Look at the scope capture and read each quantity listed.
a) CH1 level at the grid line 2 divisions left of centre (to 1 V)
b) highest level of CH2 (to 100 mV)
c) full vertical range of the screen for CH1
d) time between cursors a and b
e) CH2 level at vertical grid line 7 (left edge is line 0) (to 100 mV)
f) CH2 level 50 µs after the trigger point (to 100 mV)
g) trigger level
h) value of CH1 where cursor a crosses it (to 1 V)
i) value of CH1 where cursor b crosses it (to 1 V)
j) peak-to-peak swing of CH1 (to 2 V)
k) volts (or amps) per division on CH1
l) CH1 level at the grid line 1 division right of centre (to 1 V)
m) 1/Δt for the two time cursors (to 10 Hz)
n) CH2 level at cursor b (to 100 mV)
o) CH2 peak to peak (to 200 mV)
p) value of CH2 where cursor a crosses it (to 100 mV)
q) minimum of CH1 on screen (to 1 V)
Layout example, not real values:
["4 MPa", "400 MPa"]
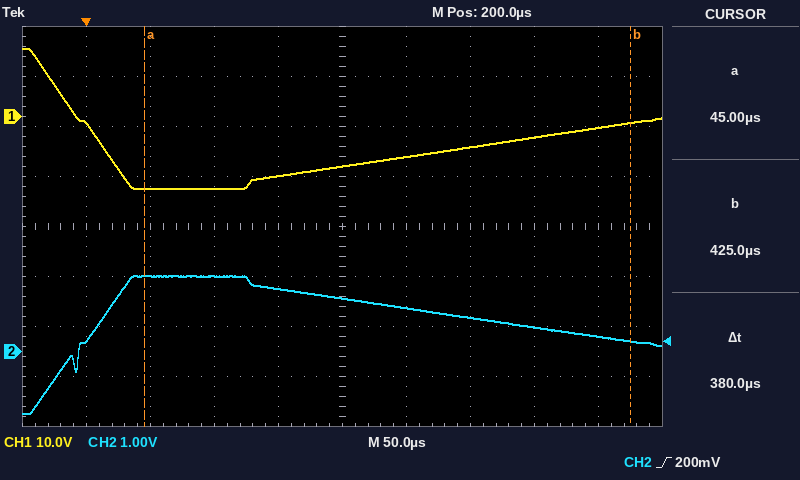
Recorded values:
["-14 V", "1.5 V", "80 V", "380 µs", "700 mV", "1.5 V", "200 mV", "-14 V", "-1 V", "28 V", "10 V", "-8 V", "2.63 kHz", "200 mV", "2.8 V", "1.5 V", "-14 V"]
